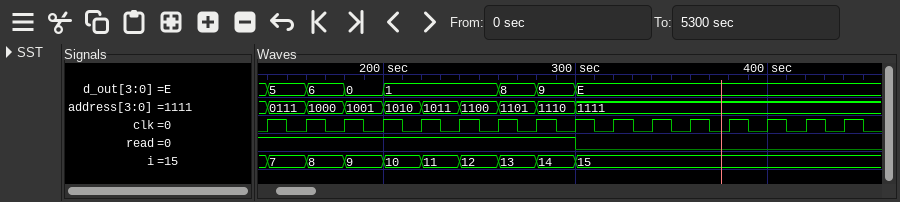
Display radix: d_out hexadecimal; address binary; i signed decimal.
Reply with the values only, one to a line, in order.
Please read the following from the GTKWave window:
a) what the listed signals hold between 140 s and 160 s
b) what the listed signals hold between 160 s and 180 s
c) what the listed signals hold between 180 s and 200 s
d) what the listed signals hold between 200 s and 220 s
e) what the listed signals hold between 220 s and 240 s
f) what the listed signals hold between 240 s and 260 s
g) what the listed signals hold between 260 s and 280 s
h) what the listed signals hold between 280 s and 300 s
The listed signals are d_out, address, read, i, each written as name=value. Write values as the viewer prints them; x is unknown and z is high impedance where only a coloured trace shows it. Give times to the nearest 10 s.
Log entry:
d_out=5, address=0111, read=1, i=7
d_out=6, address=1000, read=1, i=8
d_out=0, address=1001, read=1, i=9
d_out=1, address=1010, read=1, i=10
d_out=1, address=1011, read=1, i=11
d_out=1, address=1100, read=1, i=12
d_out=8, address=1101, read=1, i=13
d_out=9, address=1110, read=1, i=14
